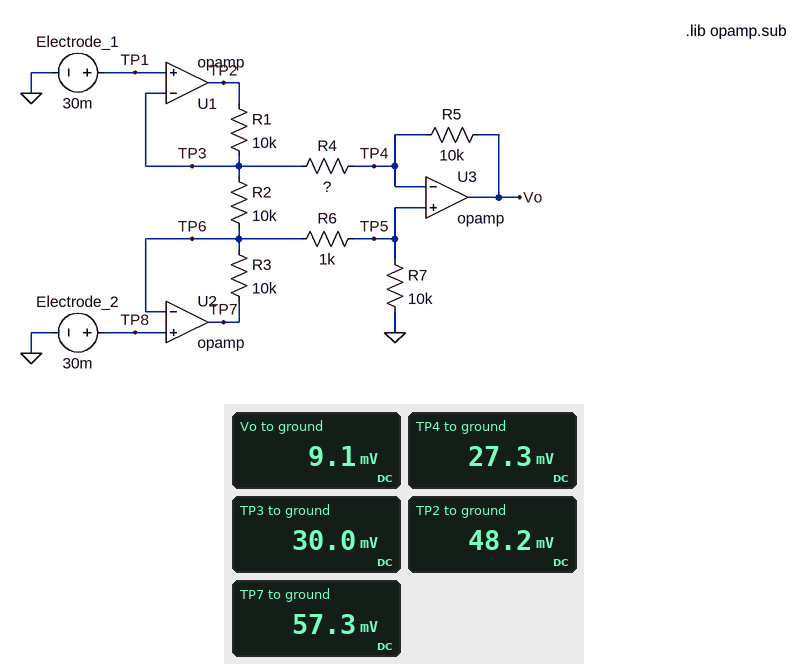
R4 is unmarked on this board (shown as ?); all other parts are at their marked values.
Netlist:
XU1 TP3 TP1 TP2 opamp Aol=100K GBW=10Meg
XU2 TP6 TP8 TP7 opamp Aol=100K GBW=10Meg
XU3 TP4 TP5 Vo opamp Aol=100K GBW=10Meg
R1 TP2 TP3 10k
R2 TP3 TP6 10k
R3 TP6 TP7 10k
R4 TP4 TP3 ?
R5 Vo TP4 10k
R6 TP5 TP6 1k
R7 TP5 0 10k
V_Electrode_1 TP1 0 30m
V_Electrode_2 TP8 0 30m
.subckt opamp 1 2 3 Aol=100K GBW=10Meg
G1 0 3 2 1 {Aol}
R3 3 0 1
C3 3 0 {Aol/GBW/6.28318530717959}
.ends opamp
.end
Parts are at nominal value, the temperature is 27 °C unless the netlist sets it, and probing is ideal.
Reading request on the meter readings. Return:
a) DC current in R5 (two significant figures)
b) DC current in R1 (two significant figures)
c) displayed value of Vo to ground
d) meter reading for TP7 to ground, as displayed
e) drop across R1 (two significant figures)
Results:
1.8 µA
1.8 µA
9.1 mV
57.3 mV
18 mV
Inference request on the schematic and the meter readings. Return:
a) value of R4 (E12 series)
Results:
1.5 kΩ
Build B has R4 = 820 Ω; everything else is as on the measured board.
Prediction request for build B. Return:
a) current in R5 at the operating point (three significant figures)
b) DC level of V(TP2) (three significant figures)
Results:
3.33 µA
63.3 mV
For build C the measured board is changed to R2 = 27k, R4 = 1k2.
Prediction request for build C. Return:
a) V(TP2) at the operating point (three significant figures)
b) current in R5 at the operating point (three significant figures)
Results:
52.7 mV
2.27 µA
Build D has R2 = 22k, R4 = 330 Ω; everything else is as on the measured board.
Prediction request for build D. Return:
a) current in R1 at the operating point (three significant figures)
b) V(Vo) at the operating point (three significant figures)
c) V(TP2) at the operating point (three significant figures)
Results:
8.26 µA
-55.3 mV
113 mV
